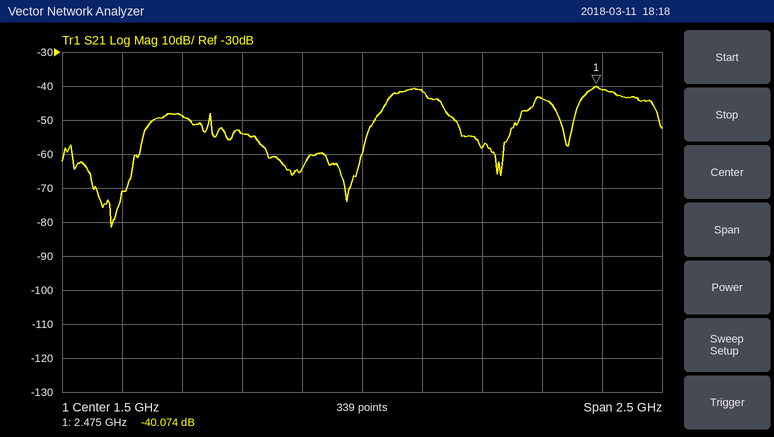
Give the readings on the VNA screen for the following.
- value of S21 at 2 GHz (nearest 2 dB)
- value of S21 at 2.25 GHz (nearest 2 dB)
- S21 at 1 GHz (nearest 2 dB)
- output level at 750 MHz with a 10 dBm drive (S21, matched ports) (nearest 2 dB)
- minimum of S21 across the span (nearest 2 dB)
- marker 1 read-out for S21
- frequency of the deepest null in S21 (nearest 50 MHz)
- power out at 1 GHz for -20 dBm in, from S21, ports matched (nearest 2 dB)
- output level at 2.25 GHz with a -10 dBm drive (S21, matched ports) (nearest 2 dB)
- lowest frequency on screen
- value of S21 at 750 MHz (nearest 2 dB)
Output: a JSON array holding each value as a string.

["-58 dB", "-44 dB", "-54 dB", "-38 dBm", "-82 dB", "-40.074 dB", "450 MHz", "-74 dBm", "-54 dBm", "250 MHz", "-48 dB"]
